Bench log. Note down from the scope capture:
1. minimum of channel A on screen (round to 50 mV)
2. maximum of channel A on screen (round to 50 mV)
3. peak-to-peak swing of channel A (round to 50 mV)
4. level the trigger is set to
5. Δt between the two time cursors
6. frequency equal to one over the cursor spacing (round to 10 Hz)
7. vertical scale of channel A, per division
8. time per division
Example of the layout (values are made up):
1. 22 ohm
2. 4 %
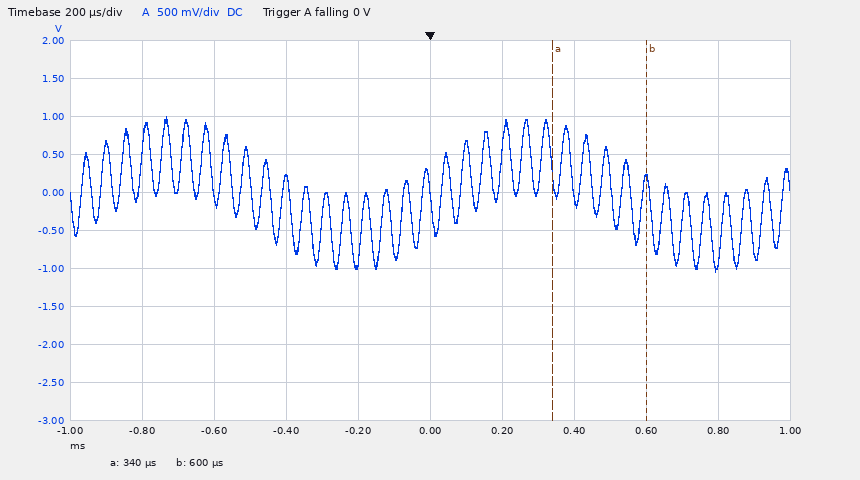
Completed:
1. -1.05 V
2. 1.00 V
3. 2.05 V
4. 0 V
5. 260 µs
6. 3.85 kHz
7. 500 mV
8. 200 µs
